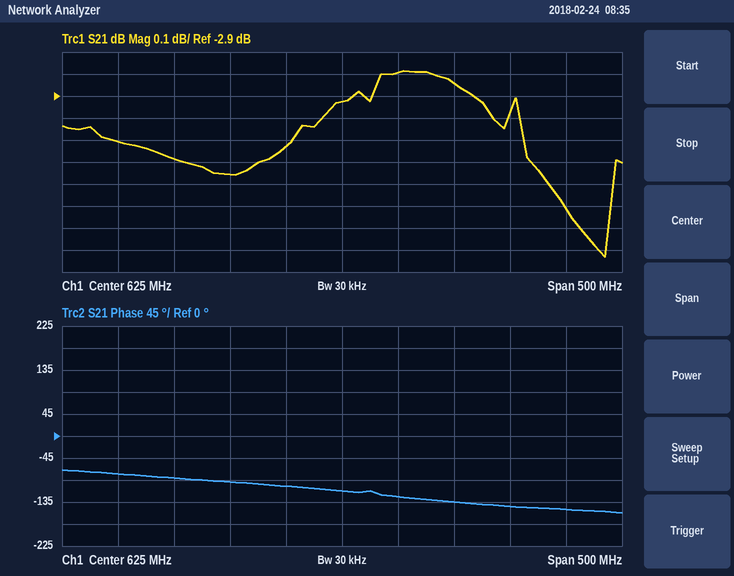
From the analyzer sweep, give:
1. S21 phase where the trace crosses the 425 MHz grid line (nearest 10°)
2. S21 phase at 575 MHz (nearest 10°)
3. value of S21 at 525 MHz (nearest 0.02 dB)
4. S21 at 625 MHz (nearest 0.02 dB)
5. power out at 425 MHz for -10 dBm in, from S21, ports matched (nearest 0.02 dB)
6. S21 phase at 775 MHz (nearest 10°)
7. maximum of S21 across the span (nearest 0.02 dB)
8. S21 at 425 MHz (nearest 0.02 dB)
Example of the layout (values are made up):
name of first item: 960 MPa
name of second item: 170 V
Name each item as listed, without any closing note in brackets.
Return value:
S21 phase where the trace crosses the 425 MHz grid line: -80°
S21 phase at 575 MHz: -100°
value of S21 at 525 MHz: -3.26 dB
S21 at 625 MHz: -2.92 dB
power out at 425 MHz for -10 dBm in, from S21, ports matched: -13.10 dBm
S21 phase at 775 MHz: -140°
maximum of S21 across the span: -2.78 dB
S21 at 425 MHz: -3.10 dB
